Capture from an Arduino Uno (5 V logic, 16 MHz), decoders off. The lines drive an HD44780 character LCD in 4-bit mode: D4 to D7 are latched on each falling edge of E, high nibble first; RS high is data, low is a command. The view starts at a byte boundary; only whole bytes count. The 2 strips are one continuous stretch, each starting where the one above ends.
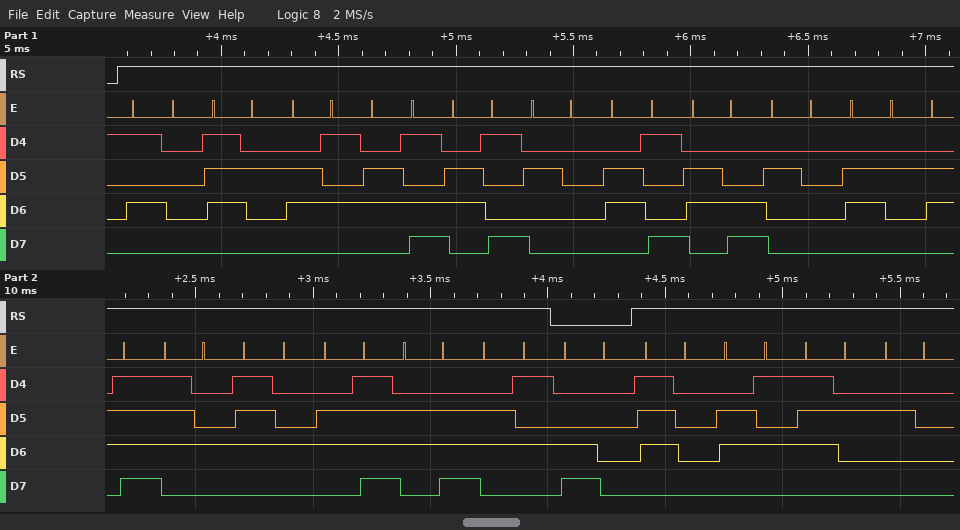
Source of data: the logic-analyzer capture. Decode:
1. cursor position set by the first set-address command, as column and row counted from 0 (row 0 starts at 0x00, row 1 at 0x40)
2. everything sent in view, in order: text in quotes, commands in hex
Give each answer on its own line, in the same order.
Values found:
column 0, row 1
"Premi il bottone" 0xC0 "per "
